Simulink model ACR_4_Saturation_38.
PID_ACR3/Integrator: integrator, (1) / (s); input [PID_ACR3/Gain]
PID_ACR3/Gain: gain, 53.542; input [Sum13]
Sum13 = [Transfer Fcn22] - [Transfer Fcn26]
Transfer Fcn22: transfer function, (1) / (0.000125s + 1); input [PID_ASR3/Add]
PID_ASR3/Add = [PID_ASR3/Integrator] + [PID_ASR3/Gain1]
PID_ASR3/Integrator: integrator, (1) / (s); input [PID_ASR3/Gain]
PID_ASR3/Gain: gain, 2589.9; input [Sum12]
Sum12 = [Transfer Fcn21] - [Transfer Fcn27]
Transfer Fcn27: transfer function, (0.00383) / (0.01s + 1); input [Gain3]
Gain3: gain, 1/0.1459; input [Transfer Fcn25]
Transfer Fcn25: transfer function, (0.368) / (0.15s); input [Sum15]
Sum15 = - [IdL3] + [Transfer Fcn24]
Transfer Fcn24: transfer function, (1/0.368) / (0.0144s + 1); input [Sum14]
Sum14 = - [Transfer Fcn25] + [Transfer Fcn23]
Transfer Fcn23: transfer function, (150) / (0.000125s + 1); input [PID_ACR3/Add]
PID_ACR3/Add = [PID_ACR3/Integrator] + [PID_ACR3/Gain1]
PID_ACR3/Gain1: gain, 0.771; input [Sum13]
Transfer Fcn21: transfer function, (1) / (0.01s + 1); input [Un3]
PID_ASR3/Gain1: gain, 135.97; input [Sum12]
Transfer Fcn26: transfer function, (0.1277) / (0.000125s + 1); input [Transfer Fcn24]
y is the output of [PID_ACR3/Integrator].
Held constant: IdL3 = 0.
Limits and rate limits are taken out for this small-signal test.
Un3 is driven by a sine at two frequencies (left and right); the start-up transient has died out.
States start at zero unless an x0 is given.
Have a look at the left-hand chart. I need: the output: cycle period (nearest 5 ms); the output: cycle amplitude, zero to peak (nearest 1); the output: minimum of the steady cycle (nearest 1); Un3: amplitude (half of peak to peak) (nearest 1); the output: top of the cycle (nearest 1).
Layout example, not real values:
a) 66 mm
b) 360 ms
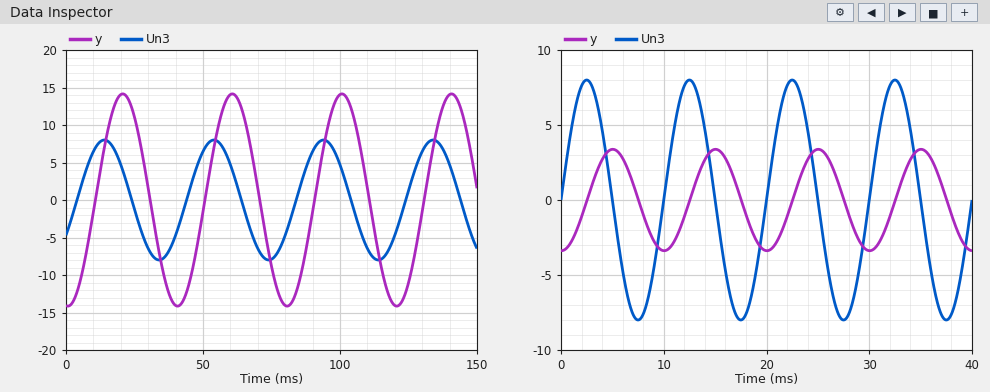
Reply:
a) 40 ms
b) 14
c) -14
d) 8
e) 14
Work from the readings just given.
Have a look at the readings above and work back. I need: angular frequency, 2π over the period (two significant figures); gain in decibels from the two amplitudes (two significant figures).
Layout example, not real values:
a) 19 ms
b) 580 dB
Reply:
a) 0.16 rad/ms
b) 4.9 dB
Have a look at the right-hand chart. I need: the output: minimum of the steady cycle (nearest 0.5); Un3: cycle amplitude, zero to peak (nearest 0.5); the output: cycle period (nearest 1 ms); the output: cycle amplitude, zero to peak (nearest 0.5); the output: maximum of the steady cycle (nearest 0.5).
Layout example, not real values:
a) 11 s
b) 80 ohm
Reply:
a) -3.5
b) 8.0
c) 10 ms
d) 3.5
e) 3.5
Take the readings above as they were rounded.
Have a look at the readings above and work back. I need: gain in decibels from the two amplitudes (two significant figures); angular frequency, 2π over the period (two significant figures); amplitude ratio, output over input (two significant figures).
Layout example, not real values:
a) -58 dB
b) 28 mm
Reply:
a) -7.2 dB
b) 0.63 rad/ms
c) 0.44
